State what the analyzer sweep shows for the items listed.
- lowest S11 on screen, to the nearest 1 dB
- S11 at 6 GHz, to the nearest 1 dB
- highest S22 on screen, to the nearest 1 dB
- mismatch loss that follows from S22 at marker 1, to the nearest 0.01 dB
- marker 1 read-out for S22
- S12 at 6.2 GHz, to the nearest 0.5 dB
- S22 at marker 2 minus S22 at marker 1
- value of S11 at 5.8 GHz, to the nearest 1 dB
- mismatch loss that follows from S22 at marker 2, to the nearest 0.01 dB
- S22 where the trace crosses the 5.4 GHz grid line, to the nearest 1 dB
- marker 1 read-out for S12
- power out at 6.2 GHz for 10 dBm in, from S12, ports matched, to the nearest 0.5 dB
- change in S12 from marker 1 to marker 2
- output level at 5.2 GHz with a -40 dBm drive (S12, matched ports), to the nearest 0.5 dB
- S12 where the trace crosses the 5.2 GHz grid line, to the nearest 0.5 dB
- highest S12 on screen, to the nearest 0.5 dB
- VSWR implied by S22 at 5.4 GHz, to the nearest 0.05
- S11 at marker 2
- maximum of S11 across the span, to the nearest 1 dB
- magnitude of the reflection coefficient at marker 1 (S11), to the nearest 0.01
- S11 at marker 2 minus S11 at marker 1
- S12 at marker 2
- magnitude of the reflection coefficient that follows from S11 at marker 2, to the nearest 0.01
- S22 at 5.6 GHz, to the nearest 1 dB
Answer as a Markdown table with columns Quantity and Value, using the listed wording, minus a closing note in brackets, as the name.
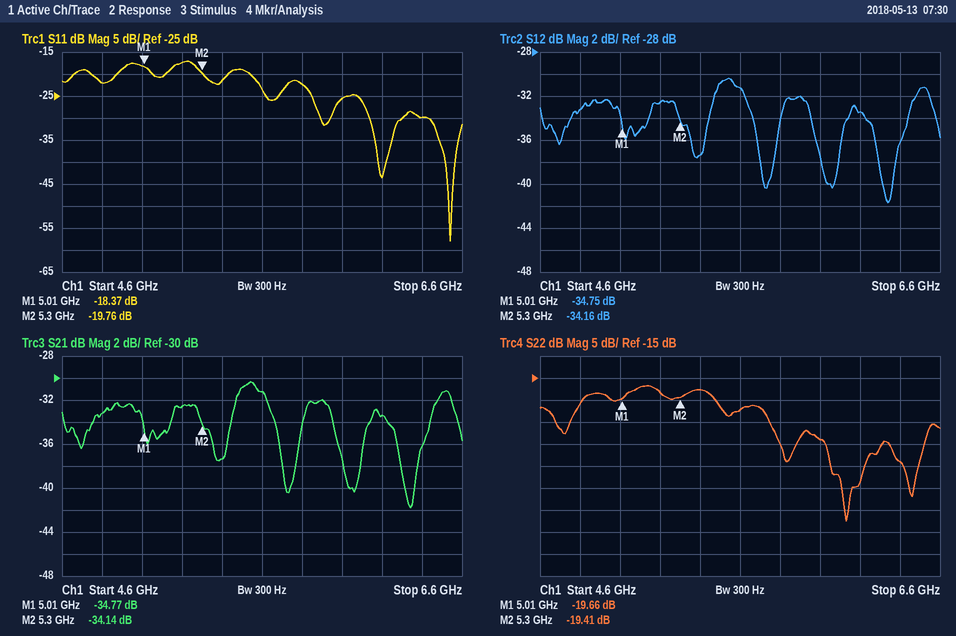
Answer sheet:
| Quantity | Value |
|---|---|
| lowest S11 on screen, to the nearest 1 dB | -58 dB |
| S11 at 6 GHz, to the nearest 1 dB | -26 dB |
| highest S22 on screen, to the nearest 1 dB | -17 dB |
| mismatch loss that follows from S22 at marker 1, to the nearest 0.01 dB | 0.05 dB |
| marker 1 read-out for S22 | -19.66 dB |
| S12 at 6.2 GHz, to the nearest 0.5 dB | -33.5 dB |
| S22 at marker 2 minus S22 at marker 1 | 0.25 dB |
| value of S11 at 5.8 GHz, to the nearest 1 dB | -22 dB |
| mismatch loss that follows from S22 at marker 2, to the nearest 0.01 dB | 0.05 dB |
| S22 where the trace crosses the 5.4 GHz grid line, to the nearest 1 dB | -18 dB |
| marker 1 read-out for S12 | -34.75 dB |
| power out at 6.2 GHz for 10 dBm in, from S12, ports matched, to the nearest 0.5 dB | -23.5 dBm |
| change in S12 from marker 1 to marker 2 | 0.59 dB |
| output level at 5.2 GHz with a -40 dBm drive (S12, matched ports), to the nearest 0.5 dB | -72.5 dBm |
| S12 where the trace crosses the 5.2 GHz grid line, to the nearest 0.5 dB | -32.5 dB |
| highest S12 on screen, to the nearest 0.5 dB | -30.5 dB |
| VSWR implied by S22 at 5.4 GHz, to the nearest 0.05 | 1.30 |
| S11 at marker 2 | -19.76 dB |
| maximum of S11 across the span, to the nearest 1 dB | -17 dB |
| magnitude of the reflection coefficient at marker 1 (S11), to the nearest 0.01 | 0.12 |
| S11 at marker 2 minus S11 at marker 1 | -1.39 dB |
| S12 at marker 2 | -34.16 dB |
| magnitude of the reflection coefficient that follows from S11 at marker 2, to the nearest 0.01 | 0.10 |
| S22 at 5.6 GHz, to the nearest 1 dB | -22 dB |
